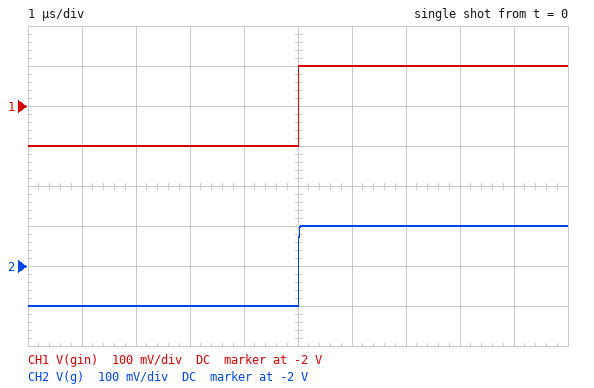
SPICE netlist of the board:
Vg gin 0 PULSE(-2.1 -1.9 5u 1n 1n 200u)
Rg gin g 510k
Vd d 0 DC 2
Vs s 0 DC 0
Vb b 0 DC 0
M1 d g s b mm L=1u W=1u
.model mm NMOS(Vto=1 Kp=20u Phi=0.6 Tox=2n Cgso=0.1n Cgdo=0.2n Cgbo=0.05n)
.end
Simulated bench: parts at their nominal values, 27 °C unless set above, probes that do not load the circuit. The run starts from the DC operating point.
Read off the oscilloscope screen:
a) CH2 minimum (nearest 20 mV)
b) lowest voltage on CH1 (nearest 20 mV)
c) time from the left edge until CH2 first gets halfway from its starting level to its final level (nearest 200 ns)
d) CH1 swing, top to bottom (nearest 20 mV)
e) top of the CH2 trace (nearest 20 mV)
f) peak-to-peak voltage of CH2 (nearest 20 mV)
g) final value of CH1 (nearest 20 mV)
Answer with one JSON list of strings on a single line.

["-2.10 V", "-2.10 V", "5.0 µs", "200 mV", "-1.90 V", "200 mV", "-1.90 V"]
